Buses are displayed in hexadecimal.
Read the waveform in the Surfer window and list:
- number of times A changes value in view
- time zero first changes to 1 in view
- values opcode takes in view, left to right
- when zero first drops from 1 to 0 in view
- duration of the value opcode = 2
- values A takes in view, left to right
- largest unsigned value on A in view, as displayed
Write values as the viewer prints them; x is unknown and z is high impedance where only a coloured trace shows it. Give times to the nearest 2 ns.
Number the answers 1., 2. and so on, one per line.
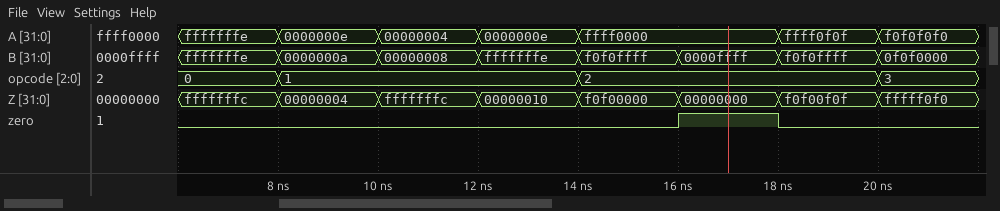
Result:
1. 6
2. 16 ns
3. 0, 1, 2, 3
4. 18 ns
5. 6 ns
6. fffffffe, 0000000e, 00000004, 0000000e, ffff0000, ffff0f0f, f0f0f0f0
7. fffffffe
